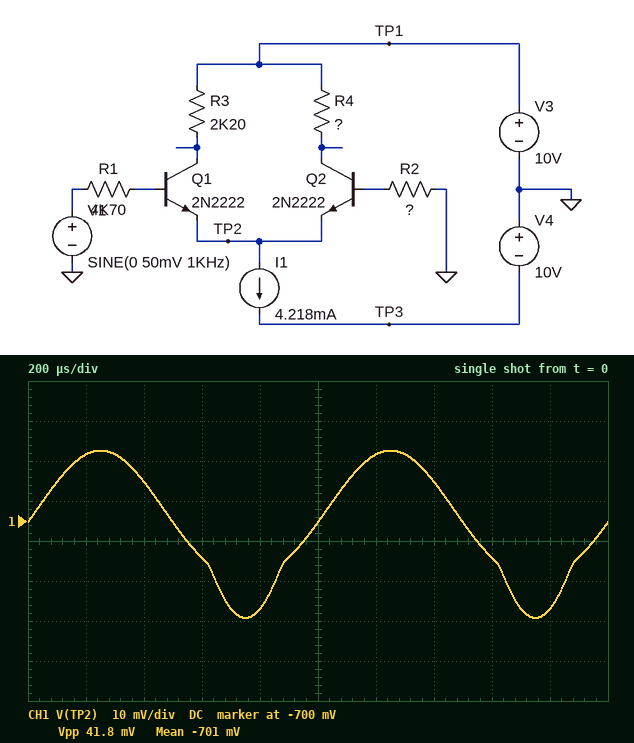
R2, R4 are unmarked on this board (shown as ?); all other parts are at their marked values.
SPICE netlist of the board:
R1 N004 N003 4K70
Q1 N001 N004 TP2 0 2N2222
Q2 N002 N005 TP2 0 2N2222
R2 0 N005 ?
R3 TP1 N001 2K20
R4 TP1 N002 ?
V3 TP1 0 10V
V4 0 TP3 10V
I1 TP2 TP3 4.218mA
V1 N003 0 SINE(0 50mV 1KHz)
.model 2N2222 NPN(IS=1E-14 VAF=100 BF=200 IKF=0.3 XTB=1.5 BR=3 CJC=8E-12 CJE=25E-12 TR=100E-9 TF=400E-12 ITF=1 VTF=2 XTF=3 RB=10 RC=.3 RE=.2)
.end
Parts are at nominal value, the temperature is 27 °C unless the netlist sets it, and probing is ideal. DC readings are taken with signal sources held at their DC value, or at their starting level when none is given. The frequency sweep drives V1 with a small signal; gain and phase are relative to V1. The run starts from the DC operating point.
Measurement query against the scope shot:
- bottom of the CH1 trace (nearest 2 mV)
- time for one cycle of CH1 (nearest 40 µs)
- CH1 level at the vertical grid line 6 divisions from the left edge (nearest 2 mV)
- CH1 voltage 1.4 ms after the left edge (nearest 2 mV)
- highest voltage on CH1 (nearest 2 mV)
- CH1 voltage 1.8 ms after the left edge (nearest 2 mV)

-724 mV
1.00 ms
-684 mV
-690 mV
-682 mV
-722 mV
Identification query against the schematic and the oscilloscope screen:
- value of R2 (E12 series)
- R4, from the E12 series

1.5 kΩ
3.3 kΩ
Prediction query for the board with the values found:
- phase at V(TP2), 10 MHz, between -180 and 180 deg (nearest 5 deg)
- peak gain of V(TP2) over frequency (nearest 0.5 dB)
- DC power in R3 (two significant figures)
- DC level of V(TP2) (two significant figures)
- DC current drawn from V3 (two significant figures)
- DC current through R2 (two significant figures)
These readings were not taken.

-30 deg
-8.0 dB
5.4 mW
-700 mV
4.2 mA
13 µA
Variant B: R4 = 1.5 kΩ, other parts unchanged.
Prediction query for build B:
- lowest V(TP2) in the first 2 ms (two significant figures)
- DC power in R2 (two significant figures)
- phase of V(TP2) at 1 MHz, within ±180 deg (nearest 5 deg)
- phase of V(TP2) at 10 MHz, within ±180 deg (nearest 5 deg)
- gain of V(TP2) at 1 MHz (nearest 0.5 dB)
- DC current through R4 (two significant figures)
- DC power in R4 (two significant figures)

-710 mV
240 nW
-10 deg
-15 deg
-14.5 dB
2.7 mA
11 mW
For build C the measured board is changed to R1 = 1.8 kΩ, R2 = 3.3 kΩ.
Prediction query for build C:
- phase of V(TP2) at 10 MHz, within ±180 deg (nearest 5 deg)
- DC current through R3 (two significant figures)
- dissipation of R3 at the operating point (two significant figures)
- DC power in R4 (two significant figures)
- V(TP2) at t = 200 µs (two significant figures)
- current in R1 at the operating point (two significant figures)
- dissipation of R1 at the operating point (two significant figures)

-20 deg
2.4 mA
13 mW
11 mW
-670 mV
12 µA
240 nW
